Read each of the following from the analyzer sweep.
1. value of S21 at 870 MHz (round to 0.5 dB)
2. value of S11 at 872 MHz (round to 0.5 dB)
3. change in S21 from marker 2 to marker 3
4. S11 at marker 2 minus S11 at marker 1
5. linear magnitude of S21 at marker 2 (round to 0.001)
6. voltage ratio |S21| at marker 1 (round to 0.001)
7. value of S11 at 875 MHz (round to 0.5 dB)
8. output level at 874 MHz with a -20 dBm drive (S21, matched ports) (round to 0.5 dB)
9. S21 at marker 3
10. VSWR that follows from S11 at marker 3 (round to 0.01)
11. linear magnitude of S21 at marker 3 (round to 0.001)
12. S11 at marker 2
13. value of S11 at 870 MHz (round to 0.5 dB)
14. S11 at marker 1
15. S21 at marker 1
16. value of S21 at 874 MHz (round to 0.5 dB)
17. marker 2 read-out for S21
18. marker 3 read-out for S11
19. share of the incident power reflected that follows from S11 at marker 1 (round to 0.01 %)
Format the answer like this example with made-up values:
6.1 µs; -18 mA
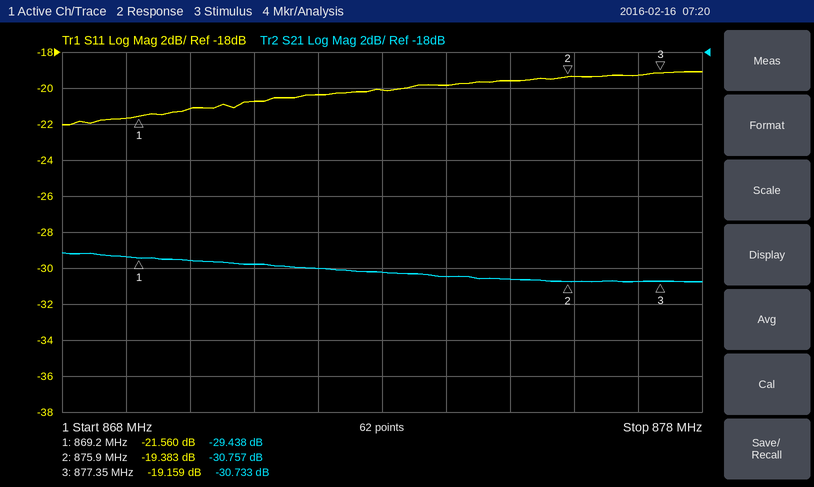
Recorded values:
-29.5 dB; -20.5 dB; 0.024 dB; 2.177 dB; 0.029; 0.034; -19.5 dB; -50.5 dBm; -30.733 dB; 1.25; 0.029; -19.383 dB; -21.0 dB; -21.560 dB; -29.438 dB; -30.5 dB; -30.757 dB; -19.159 dB; 0.70 %
